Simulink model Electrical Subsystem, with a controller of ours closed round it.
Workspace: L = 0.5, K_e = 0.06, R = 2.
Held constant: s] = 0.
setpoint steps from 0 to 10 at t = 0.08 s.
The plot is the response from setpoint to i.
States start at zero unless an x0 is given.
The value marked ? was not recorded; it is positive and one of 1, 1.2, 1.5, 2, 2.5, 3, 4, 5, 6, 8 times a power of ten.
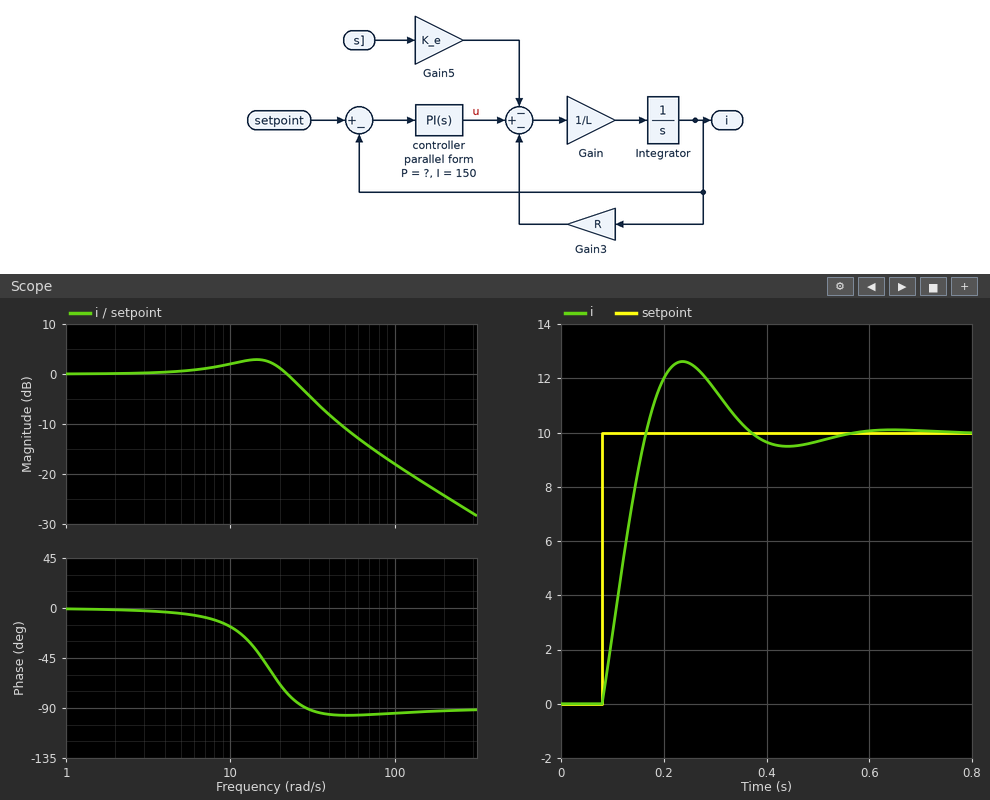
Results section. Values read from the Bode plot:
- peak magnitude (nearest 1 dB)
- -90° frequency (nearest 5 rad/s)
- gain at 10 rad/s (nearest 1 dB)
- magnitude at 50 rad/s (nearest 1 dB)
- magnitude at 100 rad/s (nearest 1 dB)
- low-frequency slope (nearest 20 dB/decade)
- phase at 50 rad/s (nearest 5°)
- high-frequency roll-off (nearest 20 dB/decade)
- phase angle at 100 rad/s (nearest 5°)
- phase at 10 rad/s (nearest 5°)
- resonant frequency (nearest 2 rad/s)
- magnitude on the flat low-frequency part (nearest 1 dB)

3 dB
30 rad/s
2 dB
-11 dB
-18 dB
0 dB/decade
-95°
-20 dB/decade
-95°
-15°
14 rad/s
0 dB
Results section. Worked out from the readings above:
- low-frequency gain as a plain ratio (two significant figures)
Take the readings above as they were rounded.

1.0
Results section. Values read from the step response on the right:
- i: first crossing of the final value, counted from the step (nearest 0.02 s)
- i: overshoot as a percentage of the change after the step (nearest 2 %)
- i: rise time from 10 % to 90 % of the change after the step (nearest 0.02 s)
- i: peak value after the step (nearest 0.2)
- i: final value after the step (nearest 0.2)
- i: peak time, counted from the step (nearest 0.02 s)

0.08 s
26 %
0.06 s
12.6
10.0
0.16 s
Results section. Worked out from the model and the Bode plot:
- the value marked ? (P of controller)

6
